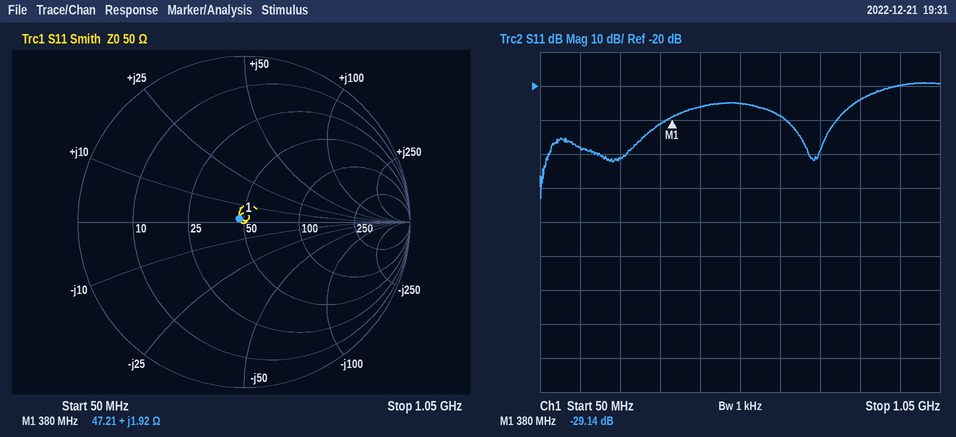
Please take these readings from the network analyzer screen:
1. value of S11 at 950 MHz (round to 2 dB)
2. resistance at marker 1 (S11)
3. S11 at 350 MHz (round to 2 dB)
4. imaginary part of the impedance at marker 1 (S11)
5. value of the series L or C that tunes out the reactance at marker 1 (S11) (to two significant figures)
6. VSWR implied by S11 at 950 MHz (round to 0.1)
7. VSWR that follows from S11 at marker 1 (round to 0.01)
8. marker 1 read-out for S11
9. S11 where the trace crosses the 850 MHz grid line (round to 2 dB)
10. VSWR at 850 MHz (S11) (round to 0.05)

-20 dB
47.21 Ω
-32 dB
+1.92 Ω
220 pF
1.2
1.07
-29.14 dB
-24 dB
1.15
